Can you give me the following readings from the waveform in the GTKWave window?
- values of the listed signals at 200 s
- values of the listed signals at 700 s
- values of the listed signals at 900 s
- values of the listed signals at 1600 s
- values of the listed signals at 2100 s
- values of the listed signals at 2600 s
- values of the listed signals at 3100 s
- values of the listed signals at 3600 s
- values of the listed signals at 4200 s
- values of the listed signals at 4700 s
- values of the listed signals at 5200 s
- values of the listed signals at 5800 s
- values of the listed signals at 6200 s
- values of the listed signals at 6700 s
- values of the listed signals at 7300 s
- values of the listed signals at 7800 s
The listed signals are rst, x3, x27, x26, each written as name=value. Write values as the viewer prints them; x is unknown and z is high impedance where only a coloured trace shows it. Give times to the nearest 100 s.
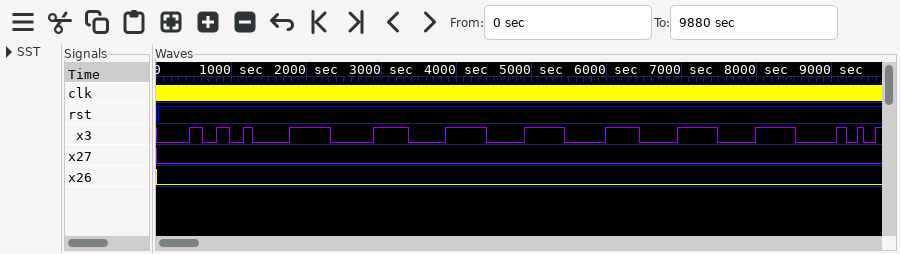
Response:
rst=1, x3=0, x27=0, x26=0
rst=1, x3=0, x27=0, x26=0
rst=1, x3=1, x27=0, x26=0
rst=1, x3=0, x27=0, x26=0
rst=1, x3=1, x27=0, x26=0
rst=1, x3=0, x27=0, x26=0
rst=1, x3=1, x27=0, x26=0
rst=1, x3=0, x27=0, x26=0
rst=1, x3=1, x27=0, x26=0
rst=1, x3=0, x27=0, x26=0
rst=1, x3=1, x27=0, x26=0
rst=1, x3=0, x27=0, x26=0
rst=1, x3=1, x27=0, x26=0
rst=1, x3=0, x27=0, x26=0
rst=1, x3=1, x27=0, x26=0
rst=1, x3=0, x27=0, x26=0
